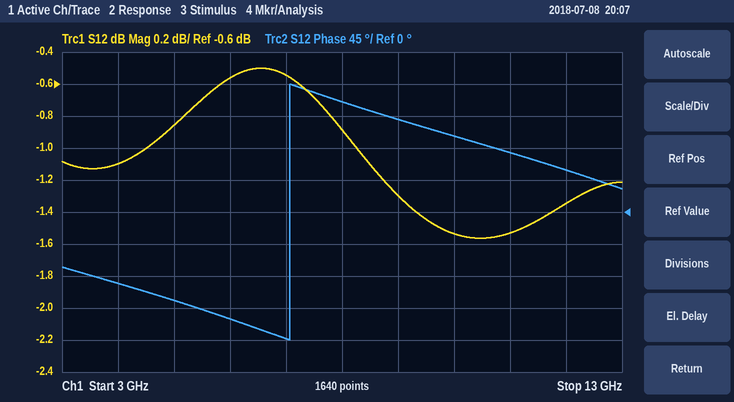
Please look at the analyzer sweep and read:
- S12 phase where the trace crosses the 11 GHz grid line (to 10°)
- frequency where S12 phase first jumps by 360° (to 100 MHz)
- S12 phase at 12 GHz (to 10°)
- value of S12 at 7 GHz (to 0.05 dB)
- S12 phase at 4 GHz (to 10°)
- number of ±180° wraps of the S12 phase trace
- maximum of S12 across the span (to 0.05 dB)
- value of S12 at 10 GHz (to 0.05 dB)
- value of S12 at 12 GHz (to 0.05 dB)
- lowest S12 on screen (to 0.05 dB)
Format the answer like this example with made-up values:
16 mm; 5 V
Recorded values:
80°; 7.1 GHz; 60°; -0.55 dB; -100°; 1; -0.50 dB; -1.55 dB; -1.35 dB; -1.55 dB
